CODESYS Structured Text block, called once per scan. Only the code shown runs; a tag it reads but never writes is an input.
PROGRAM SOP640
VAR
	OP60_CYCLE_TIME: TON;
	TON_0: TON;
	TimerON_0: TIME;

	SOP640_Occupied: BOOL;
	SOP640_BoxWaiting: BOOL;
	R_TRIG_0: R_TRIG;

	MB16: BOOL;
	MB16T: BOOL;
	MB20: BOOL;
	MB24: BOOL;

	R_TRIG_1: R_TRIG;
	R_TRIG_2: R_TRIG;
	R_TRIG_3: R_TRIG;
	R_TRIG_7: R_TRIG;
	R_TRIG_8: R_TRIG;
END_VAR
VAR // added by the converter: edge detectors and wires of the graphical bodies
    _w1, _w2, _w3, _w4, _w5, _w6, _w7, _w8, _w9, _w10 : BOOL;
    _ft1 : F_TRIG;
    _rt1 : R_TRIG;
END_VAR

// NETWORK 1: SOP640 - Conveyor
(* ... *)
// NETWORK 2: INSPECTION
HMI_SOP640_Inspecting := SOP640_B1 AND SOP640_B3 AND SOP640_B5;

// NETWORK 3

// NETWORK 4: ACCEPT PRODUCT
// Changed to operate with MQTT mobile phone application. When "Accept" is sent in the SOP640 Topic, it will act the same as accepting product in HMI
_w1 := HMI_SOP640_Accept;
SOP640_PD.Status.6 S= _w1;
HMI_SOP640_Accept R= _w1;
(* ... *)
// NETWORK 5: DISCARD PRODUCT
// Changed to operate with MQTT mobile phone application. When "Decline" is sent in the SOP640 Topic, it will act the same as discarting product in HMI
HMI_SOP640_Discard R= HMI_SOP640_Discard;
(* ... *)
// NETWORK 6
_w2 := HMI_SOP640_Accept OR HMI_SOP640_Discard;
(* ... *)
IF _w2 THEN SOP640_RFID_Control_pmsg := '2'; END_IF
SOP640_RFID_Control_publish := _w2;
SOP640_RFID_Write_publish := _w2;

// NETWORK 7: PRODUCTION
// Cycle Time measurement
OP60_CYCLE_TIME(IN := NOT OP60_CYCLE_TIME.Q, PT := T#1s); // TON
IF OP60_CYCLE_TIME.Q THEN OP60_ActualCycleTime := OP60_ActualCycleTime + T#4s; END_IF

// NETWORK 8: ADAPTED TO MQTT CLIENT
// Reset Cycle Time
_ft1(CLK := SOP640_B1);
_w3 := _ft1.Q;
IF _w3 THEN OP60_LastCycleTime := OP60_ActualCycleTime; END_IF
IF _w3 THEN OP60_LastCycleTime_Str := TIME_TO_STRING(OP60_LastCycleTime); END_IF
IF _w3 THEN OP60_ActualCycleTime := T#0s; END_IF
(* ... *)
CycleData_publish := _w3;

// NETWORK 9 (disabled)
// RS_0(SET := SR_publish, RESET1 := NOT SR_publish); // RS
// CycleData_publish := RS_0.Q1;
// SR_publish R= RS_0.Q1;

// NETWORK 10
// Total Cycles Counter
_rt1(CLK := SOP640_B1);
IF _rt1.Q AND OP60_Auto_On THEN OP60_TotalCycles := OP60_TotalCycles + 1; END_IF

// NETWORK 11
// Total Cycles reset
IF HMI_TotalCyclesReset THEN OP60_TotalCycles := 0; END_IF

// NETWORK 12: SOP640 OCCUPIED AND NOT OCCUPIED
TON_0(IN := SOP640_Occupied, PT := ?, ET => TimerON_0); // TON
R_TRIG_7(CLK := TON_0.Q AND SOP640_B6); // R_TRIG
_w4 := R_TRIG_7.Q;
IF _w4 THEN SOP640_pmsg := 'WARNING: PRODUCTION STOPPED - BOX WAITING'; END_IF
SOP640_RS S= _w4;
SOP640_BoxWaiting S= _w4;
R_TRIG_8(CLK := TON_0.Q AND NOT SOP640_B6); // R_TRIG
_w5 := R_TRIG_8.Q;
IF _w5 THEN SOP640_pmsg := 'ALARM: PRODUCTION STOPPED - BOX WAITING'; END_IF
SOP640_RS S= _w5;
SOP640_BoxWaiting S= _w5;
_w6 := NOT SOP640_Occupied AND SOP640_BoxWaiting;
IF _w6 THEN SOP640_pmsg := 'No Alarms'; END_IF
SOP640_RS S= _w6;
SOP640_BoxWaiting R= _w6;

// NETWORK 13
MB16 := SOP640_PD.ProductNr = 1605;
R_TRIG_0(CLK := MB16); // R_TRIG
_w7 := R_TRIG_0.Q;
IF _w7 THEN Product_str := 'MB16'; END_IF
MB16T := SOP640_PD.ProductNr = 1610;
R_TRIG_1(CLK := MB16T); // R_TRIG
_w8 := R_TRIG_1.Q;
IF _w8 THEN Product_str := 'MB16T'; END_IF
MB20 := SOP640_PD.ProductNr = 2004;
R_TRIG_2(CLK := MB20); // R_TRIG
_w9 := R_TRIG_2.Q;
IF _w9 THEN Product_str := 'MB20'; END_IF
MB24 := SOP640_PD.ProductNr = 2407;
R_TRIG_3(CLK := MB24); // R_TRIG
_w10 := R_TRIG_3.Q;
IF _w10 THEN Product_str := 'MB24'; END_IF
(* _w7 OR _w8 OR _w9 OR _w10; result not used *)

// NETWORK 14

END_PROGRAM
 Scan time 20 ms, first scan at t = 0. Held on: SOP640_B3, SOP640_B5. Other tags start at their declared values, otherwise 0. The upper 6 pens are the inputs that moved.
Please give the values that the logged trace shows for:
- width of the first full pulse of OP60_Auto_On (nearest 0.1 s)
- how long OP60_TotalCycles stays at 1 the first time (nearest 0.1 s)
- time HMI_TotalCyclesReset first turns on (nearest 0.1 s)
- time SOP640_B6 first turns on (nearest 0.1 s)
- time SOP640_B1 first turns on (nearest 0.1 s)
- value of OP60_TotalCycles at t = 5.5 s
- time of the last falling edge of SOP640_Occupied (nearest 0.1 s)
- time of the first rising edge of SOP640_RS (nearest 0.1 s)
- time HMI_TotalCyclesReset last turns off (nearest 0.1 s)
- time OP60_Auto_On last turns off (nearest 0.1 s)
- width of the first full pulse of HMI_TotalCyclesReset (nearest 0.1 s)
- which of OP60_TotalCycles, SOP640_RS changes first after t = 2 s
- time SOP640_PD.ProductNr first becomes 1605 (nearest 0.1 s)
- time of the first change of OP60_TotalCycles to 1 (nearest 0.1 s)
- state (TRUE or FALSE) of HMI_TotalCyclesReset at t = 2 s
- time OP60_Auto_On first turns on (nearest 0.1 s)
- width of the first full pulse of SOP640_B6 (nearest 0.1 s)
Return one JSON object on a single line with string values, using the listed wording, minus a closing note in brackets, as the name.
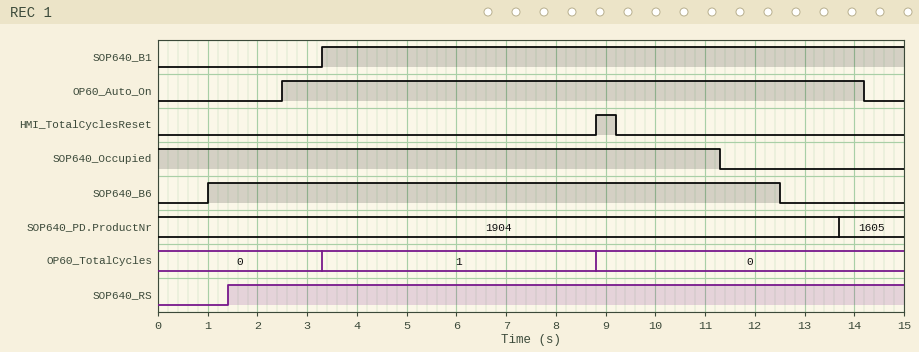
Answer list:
{"width of the first full pulse of OP60_Auto_On": "11.7 s", "how long OP60_TotalCycles stays at 1 the first time": "5.5 s", "time HMI_TotalCyclesReset first turns on": "8.8 s", "time SOP640_B6 first turns on": "1.0 s", "time SOP640_B1 first turns on": "3.3 s", "value of OP60_TotalCycles at t = 5.5 s": "1", "time of the last falling edge of SOP640_Occupied": "11.3 s", "time of the first rising edge of SOP640_RS": "1.4 s", "time HMI_TotalCyclesReset last turns off": "9.2 s", "time OP60_Auto_On last turns off": "14.2 s", "width of the first full pulse of HMI_TotalCyclesReset": "0.4 s", "which of OP60_TotalCycles, SOP640_RS changes first after t = 2 s": "OP60_TotalCycles", "time SOP640_PD.ProductNr first becomes 1605": "13.7 s", "time of the first change of OP60_TotalCycles to 1": "3.3 s", "state (TRUE or FALSE) of HMI_TotalCyclesReset at t = 2 s": "FALSE", "time OP60_Auto_On first turns on": "2.5 s", "width of the first full pulse of SOP640_B6": "11.5 s"}
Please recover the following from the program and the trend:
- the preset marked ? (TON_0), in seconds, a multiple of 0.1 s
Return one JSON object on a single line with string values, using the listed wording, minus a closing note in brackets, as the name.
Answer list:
{"the preset marked ? (TON_0), in seconds, a multiple of 0.1 s": "1.4 s"}
